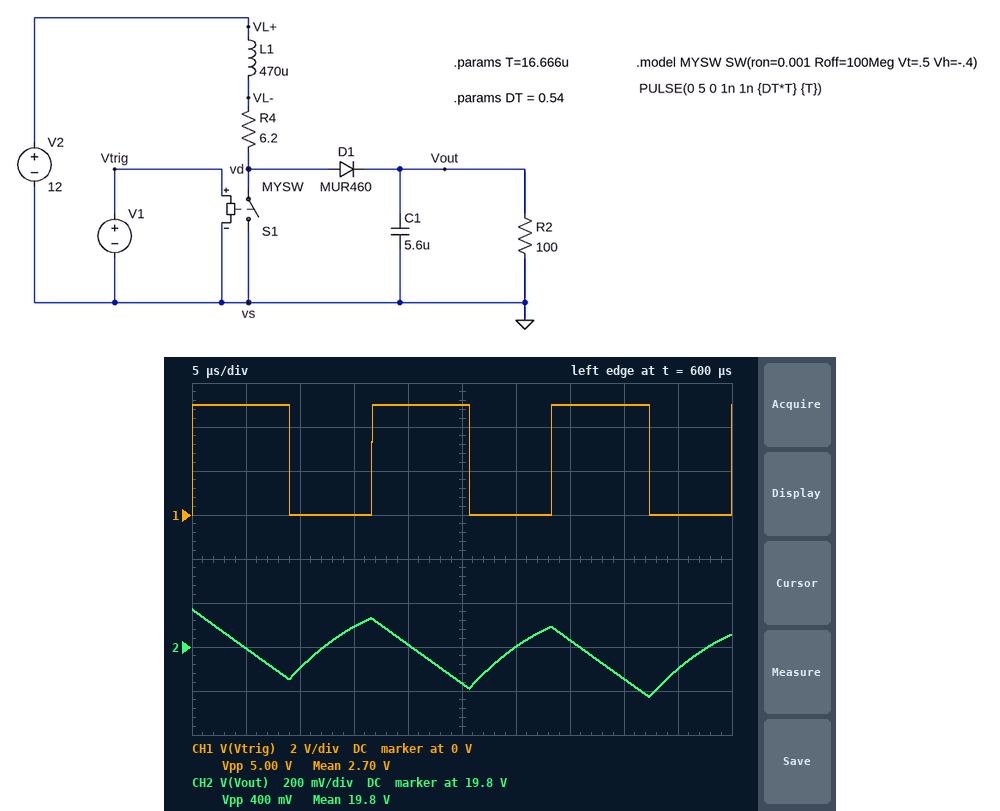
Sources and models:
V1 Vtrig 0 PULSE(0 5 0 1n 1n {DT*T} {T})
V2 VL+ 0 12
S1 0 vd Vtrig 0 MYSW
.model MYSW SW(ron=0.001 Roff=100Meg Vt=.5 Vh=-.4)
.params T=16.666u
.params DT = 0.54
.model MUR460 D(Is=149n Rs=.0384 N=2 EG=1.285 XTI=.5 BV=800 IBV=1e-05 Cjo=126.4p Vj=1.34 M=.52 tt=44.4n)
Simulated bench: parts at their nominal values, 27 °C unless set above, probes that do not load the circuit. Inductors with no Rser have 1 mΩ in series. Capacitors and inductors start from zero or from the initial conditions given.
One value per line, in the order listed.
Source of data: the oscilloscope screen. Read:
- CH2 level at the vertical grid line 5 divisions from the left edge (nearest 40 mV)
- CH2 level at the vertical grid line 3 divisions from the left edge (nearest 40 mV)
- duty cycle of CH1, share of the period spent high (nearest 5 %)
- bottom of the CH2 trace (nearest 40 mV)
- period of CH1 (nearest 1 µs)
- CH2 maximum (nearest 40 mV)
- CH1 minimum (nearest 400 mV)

19.64 V
19.88 V
55 %
19.56 V
17 µs
19.96 V
0 V
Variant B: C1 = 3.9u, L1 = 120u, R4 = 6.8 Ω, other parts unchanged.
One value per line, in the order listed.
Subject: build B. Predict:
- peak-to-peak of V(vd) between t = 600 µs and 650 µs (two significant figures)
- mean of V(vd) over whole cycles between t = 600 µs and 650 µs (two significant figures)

20 V
9.0 V
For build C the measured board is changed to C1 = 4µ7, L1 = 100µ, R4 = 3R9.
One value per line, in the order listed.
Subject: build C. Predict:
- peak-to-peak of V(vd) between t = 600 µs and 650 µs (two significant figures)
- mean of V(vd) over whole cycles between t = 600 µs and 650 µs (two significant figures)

22 V
10 V
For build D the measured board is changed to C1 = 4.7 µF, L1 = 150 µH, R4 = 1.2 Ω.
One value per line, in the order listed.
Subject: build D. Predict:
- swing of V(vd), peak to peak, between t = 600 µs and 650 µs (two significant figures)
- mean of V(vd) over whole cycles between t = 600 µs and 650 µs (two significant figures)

25 V
11 V
